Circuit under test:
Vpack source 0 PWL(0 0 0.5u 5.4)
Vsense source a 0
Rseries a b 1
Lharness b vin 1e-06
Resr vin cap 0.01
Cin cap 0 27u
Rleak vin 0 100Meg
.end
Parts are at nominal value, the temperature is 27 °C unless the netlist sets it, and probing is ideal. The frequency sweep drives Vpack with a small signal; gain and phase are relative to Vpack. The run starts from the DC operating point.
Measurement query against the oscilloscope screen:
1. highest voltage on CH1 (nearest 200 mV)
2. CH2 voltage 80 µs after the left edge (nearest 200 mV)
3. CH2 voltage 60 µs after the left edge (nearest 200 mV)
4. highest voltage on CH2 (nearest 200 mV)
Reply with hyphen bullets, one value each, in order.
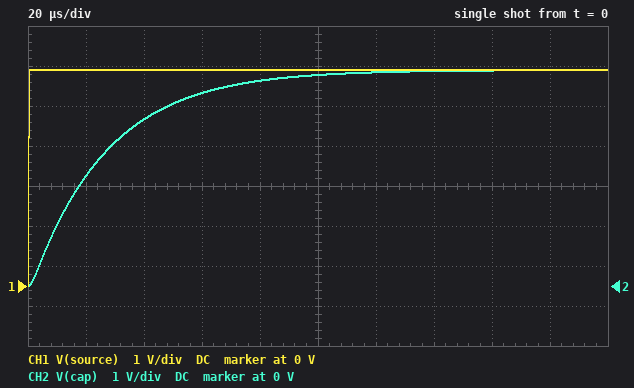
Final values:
- 5.4 V
- 5.2 V
- 4.8 V
- 5.4 V
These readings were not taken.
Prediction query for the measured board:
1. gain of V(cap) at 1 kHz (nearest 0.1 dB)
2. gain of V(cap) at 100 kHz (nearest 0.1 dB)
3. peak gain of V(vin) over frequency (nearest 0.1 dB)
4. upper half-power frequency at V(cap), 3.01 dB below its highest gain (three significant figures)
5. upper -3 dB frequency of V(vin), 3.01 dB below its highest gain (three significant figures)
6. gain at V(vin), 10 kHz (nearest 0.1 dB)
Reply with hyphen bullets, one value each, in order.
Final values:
- -0.1 dB
- -25.9 dB
- 0 dB
- 6.06 kHz
- 6.06 kHz
- -5.7 dB
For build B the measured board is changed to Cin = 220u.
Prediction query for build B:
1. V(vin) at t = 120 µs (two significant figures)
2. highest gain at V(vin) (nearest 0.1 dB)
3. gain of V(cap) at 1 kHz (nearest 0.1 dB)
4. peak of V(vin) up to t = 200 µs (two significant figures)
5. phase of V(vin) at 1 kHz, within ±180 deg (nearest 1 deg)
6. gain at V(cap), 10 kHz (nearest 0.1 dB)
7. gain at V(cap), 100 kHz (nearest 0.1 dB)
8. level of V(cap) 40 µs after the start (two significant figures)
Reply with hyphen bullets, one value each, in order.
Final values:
- 2.3 V
- 0 dB
- -4.7 dB
- 3.2 V
- -54 deg
- -22.9 dB
- -44.3 dB
- 870 mV
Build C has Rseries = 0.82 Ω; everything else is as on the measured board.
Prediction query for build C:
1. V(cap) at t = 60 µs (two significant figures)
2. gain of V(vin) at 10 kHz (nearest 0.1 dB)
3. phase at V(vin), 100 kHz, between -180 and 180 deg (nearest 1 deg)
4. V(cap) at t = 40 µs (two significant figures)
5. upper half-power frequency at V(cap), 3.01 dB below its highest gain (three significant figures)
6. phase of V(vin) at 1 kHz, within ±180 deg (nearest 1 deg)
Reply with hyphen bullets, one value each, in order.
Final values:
- 5.1 V
- -4.4 dB
- -115 deg
- 4.5 V
- 7.50 kHz
- -8 deg
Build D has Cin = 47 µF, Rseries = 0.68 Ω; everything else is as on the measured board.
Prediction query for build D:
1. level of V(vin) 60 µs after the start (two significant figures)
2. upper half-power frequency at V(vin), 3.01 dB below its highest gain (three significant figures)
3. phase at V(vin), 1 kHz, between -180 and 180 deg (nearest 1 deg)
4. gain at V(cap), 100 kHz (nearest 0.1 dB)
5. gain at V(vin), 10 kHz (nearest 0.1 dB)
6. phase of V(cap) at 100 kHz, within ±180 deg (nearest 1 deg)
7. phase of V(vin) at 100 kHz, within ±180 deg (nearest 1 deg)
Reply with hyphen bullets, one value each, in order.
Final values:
- 4.6 V
- 5.14 kHz
- -11 deg
- -28.6 dB
- -6.8 dB
- -131 deg
- -114 deg
